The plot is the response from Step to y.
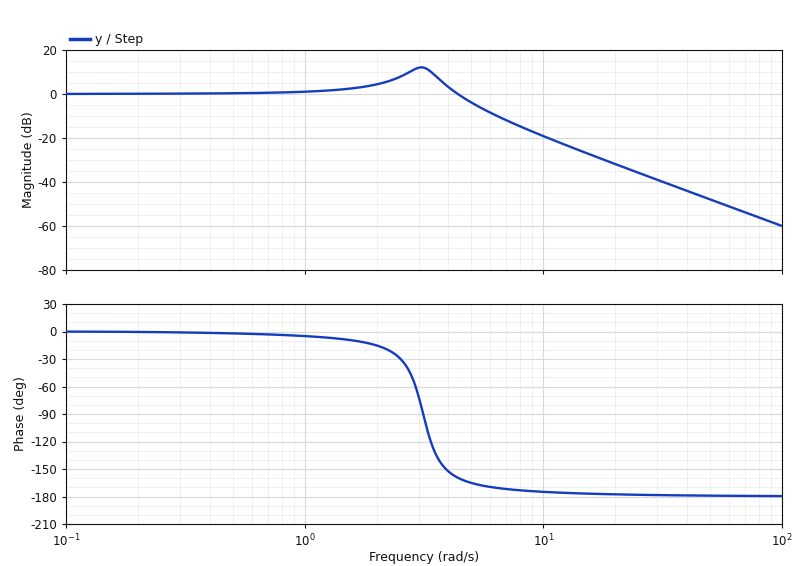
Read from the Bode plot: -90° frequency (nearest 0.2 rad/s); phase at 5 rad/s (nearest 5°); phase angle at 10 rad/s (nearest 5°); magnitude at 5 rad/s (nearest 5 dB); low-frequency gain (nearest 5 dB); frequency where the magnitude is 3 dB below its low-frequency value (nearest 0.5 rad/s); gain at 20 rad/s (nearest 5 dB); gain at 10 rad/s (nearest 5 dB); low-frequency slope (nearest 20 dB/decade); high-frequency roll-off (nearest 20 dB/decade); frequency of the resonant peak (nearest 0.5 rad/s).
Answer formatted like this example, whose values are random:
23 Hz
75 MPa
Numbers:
3.2 rad/s
-165°
-175°
-5 dB
0 dB
5.0 rad/s
-30 dB
-20 dB
0 dB/decade
-40 dB/decade
3.0 rad/s
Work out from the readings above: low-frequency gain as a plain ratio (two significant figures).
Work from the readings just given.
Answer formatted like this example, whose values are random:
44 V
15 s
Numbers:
1.0
